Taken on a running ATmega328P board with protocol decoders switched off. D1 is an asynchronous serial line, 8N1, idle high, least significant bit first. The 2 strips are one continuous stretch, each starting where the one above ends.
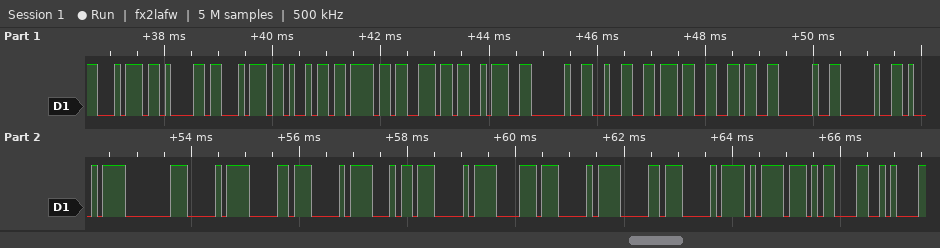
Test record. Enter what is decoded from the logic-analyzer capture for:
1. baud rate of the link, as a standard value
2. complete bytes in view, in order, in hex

9600 baud
74 61 74 69 6F 6E 3A 20 32 37 36 20 20 D1 80 D0 B0 D0 B4 D0 B8 D0 B0 D0 BD 0D 0A
